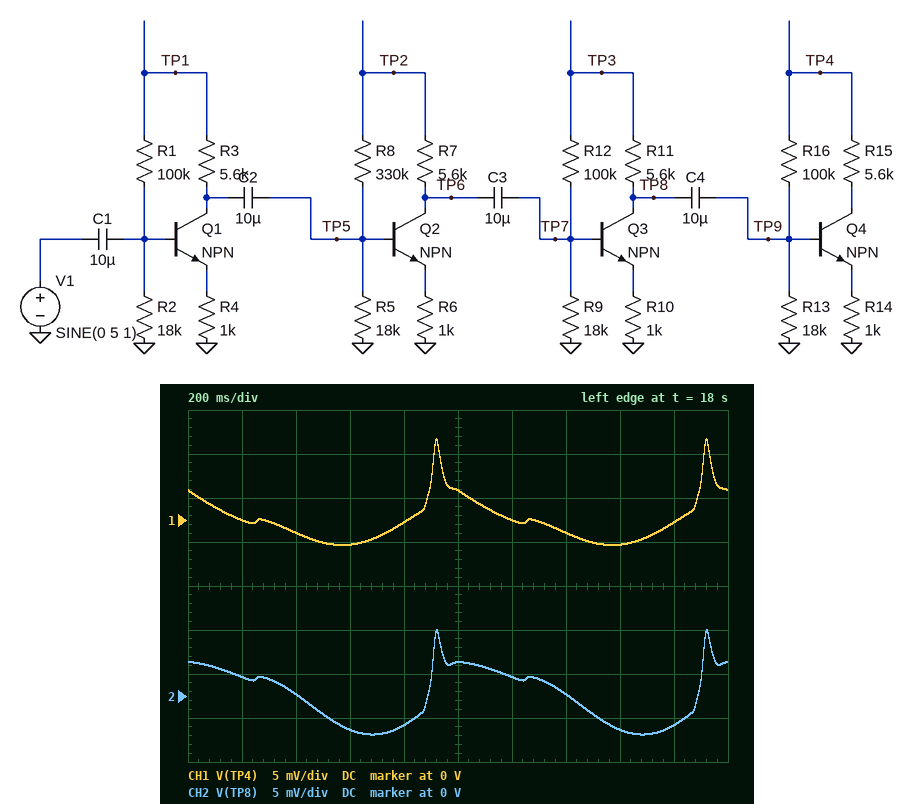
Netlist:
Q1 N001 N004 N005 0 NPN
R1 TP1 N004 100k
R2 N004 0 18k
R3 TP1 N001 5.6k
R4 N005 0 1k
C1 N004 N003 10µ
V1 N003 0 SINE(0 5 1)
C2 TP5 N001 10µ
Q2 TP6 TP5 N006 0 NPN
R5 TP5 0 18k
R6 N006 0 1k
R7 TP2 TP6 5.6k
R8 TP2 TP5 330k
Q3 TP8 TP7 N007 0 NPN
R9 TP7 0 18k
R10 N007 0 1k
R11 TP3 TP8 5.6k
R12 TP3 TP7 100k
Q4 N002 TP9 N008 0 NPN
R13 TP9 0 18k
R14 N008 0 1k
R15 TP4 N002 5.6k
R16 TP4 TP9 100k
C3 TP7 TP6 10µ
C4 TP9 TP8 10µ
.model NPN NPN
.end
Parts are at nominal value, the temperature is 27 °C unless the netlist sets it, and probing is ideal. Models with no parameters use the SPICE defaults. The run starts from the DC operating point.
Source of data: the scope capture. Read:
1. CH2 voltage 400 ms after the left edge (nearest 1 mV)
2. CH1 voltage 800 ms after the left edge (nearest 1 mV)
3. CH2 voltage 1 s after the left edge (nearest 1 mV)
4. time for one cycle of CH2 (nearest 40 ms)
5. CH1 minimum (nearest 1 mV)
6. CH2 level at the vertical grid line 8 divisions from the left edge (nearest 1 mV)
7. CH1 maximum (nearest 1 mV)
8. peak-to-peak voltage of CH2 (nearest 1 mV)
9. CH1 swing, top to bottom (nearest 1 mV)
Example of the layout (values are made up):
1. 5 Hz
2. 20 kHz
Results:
1. 0 V
2. 0 V
3. 4 mV
4. 1.00 s
5. -3 mV
6. -4 mV
7. 9 mV
8. 12 mV
9. 12 mV
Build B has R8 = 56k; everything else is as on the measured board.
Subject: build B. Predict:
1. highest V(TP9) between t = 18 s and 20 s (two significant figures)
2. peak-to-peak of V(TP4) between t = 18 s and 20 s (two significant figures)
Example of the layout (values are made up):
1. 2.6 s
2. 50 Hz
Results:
1. 20 mV
2. 30 mV
